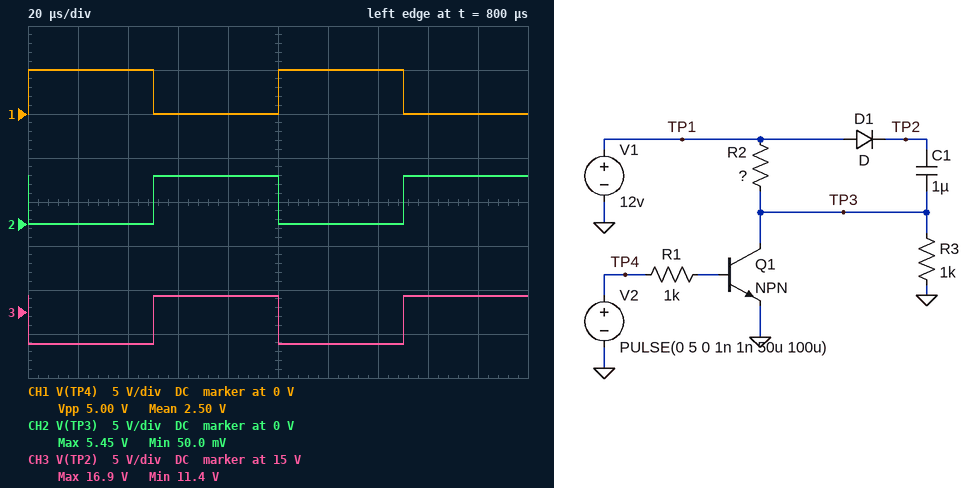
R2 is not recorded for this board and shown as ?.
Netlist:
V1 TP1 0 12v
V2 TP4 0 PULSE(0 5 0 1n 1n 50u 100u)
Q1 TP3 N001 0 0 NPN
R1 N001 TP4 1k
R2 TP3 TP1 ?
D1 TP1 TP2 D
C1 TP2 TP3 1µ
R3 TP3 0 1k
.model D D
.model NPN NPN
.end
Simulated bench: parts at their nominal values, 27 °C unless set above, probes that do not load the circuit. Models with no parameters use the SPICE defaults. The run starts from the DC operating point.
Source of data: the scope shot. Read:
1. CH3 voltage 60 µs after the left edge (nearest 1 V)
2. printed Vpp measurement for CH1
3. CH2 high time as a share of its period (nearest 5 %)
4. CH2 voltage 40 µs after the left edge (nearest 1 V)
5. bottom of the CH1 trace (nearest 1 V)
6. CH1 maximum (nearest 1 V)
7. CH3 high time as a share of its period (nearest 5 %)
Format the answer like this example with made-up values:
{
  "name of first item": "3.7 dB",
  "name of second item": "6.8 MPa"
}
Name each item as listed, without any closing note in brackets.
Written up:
{
  "CH3 voltage 60 µs after the left edge": "17 V",
  "printed Vpp measurement for CH1": "5.00 V",
  "CH2 high time as a share of its period": "50 %",
  "CH2 voltage 40 µs after the left edge": "0 V",
  "bottom of the CH1 trace": "0 V",
  "CH1 maximum": "5 V",
  "CH3 high time as a share of its period": "50 %"
}
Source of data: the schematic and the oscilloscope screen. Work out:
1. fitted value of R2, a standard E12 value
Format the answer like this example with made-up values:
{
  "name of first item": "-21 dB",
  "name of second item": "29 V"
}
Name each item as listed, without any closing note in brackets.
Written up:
{
  "fitted value of R2, a standard E12 value": "1.2 kΩ"
}
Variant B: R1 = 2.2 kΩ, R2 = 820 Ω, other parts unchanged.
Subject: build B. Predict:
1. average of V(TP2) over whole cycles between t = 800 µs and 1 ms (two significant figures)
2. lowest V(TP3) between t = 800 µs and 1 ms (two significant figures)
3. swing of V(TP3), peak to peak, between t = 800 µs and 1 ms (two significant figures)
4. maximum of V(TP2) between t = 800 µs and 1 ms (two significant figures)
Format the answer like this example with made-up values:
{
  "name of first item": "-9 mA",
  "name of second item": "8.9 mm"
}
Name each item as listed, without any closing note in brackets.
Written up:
{
  "average of V(TP2) over whole cycles between t = 800 µs and 1 ms": "15 V",
  "lowest V(TP3) between t = 800 µs and 1 ms": "61 mV",
  "swing of V(TP3), peak to peak, between t = 800 µs and 1 ms": "6.5 V",
  "maximum of V(TP2) between t = 800 µs and 1 ms": "18 V"
}
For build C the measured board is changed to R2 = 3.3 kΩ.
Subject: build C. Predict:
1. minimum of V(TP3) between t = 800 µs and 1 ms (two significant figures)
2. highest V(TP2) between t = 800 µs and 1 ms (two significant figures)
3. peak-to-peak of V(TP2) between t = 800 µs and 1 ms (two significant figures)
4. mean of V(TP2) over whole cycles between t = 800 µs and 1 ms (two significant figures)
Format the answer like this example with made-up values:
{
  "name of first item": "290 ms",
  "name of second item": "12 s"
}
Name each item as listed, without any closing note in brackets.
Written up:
{
  "minimum of V(TP3) between t = 800 µs and 1 ms": "28 mV",
  "highest V(TP2) between t = 800 µs and 1 ms": "14 V",
  "peak-to-peak of V(TP2) between t = 800 µs and 1 ms": "2.8 V",
  "mean of V(TP2) over whole cycles between t = 800 µs and 1 ms": "13 V"
}
